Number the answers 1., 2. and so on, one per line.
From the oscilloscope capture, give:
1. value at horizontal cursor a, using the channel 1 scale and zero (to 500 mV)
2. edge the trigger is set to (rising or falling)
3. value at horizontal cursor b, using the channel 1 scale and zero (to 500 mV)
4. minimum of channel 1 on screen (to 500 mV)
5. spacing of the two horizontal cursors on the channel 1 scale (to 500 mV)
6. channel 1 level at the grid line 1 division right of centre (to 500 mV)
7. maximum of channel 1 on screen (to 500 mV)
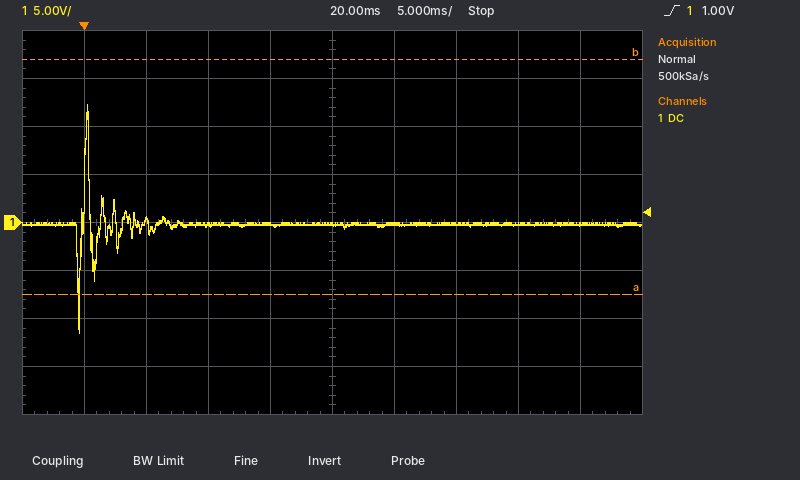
1. -7.5 V
2. rising
3. 17.0 V
4. -11.5 V
5. 24.5 V
6. 0.0 V
7. 12.5 V
